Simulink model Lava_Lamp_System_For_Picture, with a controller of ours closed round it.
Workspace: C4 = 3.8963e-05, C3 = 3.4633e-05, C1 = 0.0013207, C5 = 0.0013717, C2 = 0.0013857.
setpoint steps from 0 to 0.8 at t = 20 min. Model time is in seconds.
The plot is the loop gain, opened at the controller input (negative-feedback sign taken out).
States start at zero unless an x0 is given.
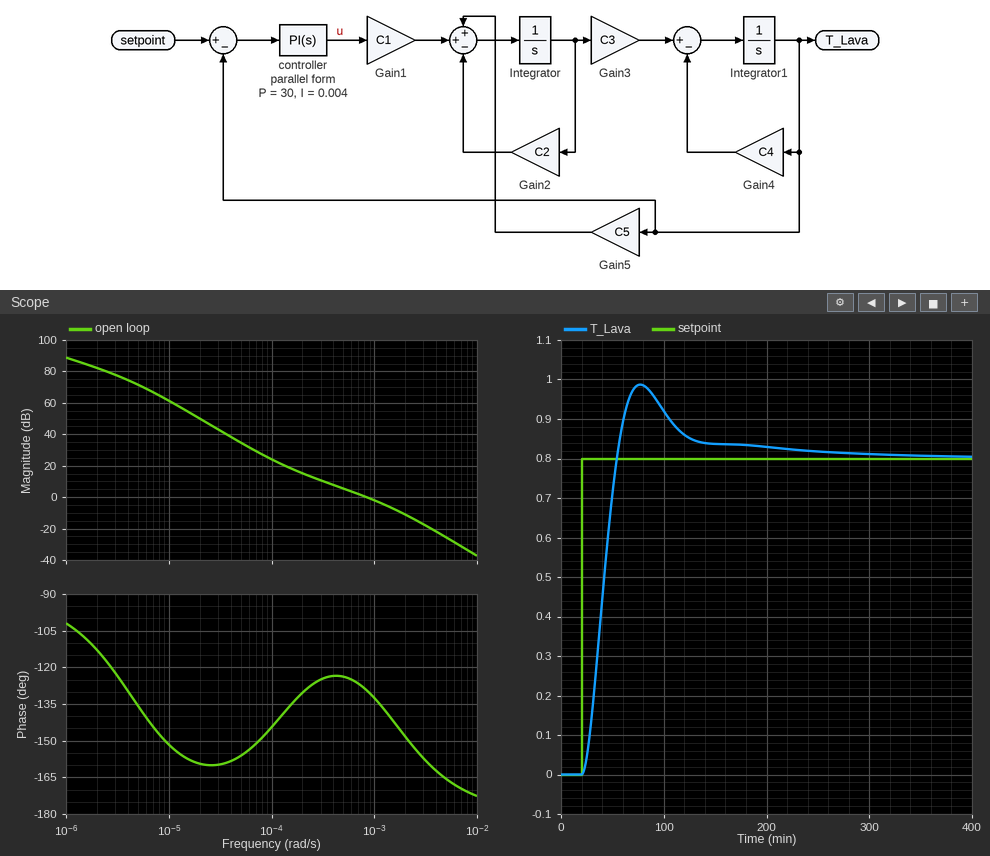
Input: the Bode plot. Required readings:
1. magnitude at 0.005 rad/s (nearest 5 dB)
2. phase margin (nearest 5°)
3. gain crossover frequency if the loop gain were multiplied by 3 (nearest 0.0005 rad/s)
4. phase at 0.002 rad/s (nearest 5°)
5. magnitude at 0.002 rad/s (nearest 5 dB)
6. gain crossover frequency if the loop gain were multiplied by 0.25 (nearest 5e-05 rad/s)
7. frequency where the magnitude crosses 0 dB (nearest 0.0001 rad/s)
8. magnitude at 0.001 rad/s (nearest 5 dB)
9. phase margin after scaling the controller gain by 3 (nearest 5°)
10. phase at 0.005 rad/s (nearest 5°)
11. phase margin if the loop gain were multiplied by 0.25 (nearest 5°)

-25 dB
50°
0.0020 rad/s
-150°
-10 dB
0.00025 rad/s
0.0008 rad/s
0 dB
35°
-165°
55°
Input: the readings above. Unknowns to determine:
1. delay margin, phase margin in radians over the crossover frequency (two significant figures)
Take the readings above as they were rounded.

1100 s
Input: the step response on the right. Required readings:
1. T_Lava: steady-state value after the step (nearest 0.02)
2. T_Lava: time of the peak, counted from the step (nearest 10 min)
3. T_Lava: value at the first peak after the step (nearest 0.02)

0.80
60 min
0.98
